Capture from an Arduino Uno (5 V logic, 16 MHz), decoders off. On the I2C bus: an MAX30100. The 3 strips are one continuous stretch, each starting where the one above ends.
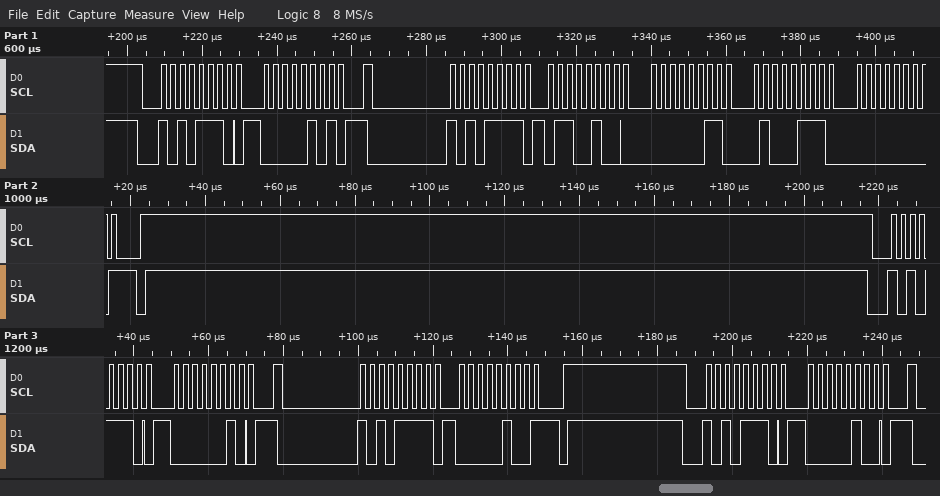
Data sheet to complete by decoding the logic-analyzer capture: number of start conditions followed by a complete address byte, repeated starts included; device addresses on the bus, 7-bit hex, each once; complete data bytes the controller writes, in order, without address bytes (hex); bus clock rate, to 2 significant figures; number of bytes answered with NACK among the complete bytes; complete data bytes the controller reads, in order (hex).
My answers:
5
0x57
05 02 04
400 kHz
2
64 03 47 00 04
